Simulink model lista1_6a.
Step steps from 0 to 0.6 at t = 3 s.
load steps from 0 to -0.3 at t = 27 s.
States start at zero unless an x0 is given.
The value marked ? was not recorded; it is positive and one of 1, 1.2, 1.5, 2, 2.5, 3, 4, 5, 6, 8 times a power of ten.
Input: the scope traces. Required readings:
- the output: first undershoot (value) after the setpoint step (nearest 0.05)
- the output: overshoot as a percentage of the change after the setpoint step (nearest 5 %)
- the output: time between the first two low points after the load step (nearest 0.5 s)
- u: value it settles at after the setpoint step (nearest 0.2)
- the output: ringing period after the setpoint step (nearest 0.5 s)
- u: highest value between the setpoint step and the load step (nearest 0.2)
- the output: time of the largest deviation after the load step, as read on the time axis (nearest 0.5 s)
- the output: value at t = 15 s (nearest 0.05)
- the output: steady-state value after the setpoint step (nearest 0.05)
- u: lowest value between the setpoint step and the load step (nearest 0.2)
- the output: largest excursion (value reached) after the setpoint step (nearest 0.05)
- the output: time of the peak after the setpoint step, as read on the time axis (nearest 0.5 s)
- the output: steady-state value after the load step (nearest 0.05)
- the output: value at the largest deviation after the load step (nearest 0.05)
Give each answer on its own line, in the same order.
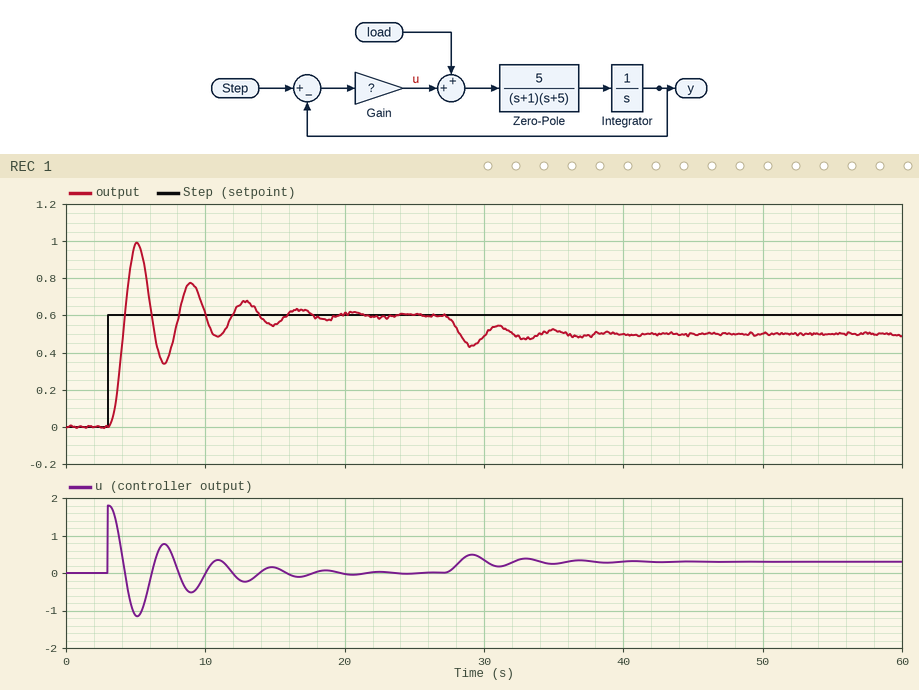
0.35
65 %
4.0 s
0.0
4.0 s
1.8
29.0 s
0.55
0.60
-1.2
1.00
5.0 s
0.50
0.45
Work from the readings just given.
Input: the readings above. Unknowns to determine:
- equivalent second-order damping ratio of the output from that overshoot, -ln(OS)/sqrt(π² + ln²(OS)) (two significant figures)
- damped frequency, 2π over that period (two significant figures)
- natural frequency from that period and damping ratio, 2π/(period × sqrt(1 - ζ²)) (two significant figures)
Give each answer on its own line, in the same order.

0.14
1.6 rad/s
1.6 rad/s
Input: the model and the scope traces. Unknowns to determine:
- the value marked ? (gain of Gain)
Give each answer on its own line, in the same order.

3
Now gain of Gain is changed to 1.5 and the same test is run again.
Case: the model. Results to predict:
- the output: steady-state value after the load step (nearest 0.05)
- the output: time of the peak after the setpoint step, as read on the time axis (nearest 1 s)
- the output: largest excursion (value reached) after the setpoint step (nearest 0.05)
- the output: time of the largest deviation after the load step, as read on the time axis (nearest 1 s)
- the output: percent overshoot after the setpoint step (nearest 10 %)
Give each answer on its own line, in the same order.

0.40
6 s
0.85
30 s
40 %
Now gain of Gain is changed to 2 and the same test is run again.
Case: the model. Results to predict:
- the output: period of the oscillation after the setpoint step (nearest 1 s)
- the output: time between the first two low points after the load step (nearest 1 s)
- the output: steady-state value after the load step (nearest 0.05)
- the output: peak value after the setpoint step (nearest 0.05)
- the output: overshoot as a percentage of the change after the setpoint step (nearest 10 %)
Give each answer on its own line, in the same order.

5 s
5 s
0.45
0.90
50 %
